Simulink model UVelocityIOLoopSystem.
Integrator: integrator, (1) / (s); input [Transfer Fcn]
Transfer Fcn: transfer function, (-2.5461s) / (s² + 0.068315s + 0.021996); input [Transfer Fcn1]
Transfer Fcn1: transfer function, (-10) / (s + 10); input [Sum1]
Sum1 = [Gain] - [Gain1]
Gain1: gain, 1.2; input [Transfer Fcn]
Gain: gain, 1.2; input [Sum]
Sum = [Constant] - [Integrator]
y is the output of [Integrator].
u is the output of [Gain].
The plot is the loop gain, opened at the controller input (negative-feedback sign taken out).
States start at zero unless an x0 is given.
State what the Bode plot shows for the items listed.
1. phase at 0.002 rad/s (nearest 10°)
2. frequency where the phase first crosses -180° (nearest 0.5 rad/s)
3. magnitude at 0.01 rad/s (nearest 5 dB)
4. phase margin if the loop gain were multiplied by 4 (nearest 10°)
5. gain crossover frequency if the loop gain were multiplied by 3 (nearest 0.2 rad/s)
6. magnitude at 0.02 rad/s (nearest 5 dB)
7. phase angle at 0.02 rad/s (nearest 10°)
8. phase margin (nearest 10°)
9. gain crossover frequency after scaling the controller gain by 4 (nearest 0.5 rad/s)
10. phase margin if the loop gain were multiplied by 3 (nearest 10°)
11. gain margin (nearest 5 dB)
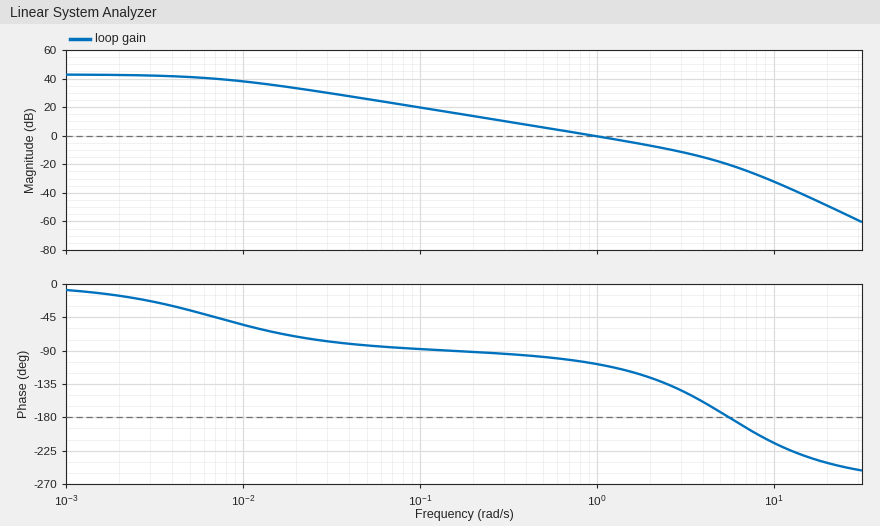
-20°
5.5 rad/s
40 dB
30°
2.6 rad/s
35 dB
-70°
70°
3.0 rad/s
40°
20 dB
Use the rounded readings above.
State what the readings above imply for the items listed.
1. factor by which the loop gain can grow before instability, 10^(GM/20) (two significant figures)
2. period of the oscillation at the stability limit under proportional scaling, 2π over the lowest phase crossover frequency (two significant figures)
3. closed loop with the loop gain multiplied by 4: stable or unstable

10
1.1 s
stable
